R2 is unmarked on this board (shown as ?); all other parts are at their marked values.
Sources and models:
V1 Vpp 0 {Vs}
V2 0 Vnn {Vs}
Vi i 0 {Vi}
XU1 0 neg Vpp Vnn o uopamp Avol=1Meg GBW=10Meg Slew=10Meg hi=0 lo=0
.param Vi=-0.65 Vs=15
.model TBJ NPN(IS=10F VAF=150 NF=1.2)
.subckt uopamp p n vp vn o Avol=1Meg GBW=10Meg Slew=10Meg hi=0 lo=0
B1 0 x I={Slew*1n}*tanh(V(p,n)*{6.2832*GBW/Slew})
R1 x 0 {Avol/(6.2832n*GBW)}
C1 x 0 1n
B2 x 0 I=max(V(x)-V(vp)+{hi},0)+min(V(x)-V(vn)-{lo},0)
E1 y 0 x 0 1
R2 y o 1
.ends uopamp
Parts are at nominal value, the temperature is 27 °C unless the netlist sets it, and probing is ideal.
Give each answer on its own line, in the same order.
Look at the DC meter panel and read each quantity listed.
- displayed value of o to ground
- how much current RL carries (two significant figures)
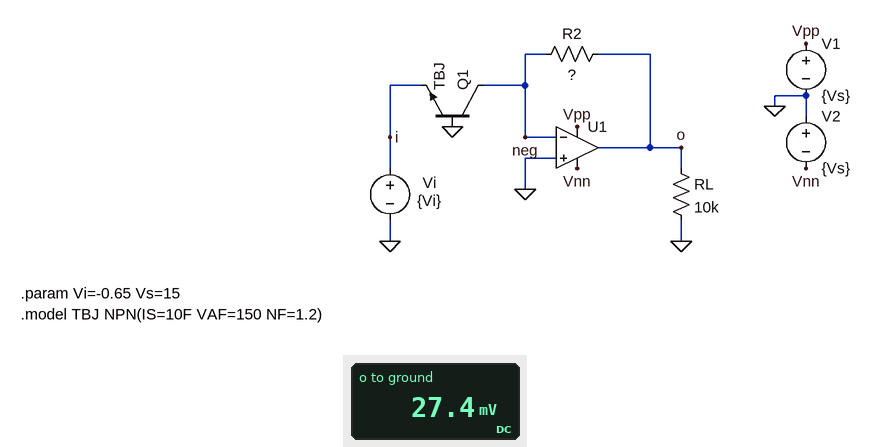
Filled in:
27.4 mV
2.7 µA
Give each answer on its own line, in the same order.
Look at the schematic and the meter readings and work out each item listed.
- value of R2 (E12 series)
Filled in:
2.2 kΩ
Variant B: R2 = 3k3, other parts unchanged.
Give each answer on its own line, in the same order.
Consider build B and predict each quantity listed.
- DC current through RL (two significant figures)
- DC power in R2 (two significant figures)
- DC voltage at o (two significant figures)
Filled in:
4.1 µA
510 nW
41 mV
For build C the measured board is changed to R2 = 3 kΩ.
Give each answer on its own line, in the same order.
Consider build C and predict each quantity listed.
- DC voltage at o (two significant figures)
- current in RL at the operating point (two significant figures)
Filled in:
37 mV
3.7 µA
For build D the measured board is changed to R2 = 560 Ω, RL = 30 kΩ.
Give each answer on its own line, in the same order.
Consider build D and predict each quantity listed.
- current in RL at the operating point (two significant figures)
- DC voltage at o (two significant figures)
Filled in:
230 nA
7.0 mV
